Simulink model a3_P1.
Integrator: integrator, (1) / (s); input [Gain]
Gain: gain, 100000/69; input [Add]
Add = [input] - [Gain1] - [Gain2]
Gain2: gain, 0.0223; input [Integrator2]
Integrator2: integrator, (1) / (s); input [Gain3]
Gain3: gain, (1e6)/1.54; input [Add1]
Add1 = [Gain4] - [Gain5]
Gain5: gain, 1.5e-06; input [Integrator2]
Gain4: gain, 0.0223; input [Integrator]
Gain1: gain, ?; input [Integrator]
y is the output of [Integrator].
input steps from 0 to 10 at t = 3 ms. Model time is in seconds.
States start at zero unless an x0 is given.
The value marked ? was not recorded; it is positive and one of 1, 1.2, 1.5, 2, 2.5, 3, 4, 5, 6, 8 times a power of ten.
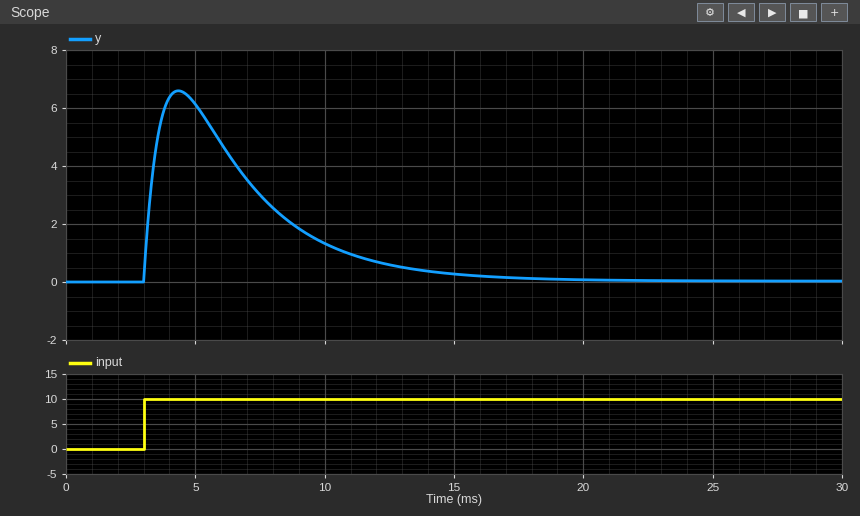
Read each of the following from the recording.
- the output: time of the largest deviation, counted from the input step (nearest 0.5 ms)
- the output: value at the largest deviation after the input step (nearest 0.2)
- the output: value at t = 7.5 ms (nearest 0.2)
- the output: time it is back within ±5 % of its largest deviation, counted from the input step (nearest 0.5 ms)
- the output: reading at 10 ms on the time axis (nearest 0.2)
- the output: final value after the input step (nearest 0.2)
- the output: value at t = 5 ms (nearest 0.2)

1.5 ms
6.6
3.0
11.0 ms
1.4
0.0
6.2
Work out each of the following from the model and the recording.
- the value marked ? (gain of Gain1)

1.2
